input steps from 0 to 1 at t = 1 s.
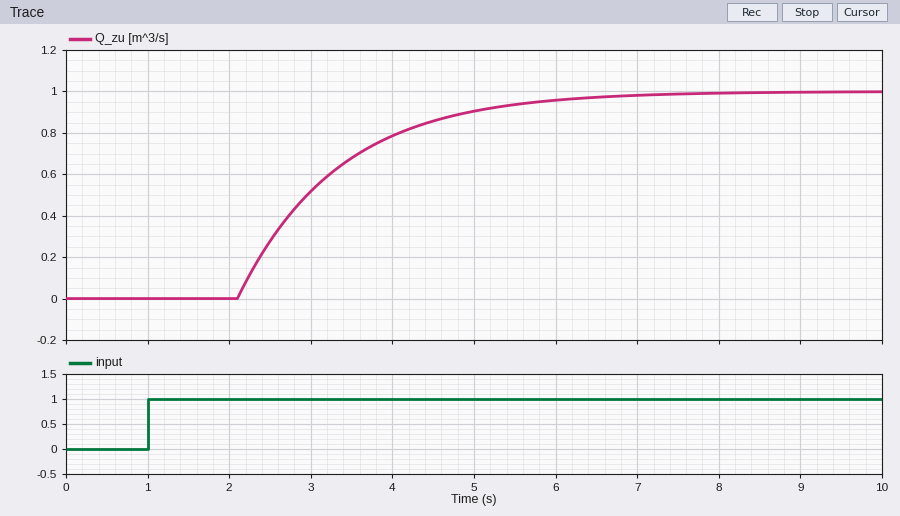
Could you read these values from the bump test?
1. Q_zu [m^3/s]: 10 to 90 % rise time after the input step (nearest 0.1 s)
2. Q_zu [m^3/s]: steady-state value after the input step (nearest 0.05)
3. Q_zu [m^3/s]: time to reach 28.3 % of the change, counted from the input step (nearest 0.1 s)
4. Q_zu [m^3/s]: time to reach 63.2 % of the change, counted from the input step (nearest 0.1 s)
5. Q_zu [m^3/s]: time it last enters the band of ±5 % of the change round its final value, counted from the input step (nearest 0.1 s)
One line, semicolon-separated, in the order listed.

2.7 s; 1.00; 1.5 s; 2.3 s; 4.8 s
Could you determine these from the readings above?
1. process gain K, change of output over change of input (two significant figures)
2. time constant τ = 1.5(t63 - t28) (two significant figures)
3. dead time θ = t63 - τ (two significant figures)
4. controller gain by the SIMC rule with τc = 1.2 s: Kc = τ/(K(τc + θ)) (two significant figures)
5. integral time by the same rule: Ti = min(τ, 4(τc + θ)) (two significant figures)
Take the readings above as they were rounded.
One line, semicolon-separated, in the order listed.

1.0; 1.2 s; 1.1 s; 0.52; 1.2 s
